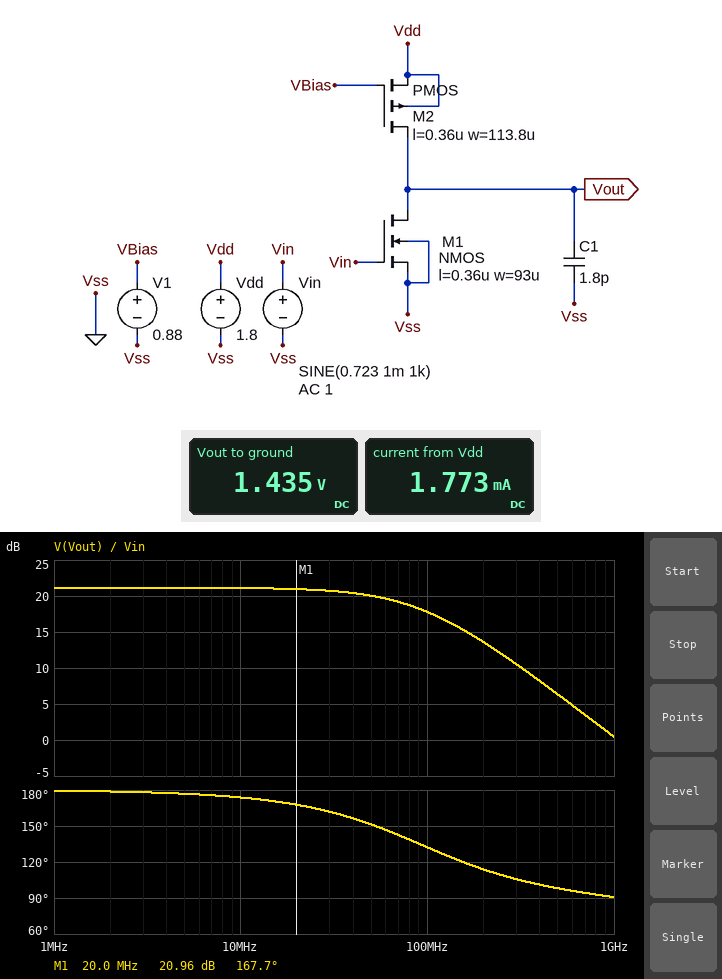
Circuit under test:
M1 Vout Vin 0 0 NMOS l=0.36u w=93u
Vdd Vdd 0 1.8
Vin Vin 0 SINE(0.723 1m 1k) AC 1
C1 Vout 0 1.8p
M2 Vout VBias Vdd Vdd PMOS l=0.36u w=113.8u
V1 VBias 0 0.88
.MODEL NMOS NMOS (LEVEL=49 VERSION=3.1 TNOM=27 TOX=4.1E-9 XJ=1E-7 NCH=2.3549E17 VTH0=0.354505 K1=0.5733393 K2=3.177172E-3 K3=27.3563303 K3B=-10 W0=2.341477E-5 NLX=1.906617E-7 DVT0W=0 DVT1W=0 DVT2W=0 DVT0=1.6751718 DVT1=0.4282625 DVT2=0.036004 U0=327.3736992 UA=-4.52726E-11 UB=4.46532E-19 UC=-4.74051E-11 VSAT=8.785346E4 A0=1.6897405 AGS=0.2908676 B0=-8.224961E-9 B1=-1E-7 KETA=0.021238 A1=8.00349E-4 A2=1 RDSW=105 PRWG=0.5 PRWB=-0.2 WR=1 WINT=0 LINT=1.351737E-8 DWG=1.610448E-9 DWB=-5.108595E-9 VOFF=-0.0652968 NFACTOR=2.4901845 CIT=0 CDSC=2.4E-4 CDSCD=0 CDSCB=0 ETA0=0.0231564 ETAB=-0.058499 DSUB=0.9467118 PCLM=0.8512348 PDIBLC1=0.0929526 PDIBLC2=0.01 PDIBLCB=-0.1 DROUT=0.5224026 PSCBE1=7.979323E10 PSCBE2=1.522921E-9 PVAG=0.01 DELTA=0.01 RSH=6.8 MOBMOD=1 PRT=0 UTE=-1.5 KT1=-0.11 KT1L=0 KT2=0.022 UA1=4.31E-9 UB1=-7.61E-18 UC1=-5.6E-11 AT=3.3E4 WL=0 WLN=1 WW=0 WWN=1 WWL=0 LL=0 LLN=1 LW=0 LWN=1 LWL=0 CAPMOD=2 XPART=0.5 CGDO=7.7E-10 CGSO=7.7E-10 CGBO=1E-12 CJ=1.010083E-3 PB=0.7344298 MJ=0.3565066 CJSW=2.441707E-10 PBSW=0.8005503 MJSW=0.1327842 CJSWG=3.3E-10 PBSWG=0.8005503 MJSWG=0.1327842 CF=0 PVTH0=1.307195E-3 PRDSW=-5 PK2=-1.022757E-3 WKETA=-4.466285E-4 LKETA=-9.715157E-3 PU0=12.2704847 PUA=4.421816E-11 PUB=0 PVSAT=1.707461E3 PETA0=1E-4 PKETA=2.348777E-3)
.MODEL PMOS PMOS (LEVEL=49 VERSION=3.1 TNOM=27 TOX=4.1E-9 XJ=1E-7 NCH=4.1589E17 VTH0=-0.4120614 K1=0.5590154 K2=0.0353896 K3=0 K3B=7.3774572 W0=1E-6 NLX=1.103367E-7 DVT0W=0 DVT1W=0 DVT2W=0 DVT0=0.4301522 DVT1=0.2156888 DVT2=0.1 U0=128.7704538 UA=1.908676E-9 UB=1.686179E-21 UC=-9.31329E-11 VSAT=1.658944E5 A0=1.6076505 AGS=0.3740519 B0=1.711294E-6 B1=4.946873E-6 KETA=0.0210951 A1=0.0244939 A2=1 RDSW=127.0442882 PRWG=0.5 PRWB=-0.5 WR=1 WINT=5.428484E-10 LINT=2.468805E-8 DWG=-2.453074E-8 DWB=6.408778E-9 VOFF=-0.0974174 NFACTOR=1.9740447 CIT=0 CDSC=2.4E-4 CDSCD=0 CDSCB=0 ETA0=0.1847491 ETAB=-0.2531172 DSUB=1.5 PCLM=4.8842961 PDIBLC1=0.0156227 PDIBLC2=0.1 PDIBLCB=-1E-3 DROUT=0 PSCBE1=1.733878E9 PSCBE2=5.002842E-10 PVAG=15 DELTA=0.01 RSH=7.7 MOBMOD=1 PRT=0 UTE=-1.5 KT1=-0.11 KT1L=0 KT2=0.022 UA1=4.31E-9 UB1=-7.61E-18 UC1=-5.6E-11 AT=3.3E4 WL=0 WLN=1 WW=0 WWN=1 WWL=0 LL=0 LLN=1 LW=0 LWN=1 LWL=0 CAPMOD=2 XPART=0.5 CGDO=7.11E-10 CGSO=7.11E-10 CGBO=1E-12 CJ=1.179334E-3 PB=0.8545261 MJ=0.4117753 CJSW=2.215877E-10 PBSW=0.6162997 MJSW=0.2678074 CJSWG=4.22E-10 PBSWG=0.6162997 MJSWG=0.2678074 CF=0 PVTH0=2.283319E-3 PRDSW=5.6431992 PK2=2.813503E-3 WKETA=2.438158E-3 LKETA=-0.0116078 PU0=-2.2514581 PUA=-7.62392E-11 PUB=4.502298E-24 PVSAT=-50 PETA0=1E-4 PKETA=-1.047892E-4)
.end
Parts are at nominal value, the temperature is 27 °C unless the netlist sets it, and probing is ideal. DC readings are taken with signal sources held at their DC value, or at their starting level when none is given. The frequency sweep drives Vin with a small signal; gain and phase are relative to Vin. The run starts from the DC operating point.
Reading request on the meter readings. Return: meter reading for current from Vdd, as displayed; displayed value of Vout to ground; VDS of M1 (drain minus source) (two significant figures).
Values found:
1.773 mA
1.435 V
1.4 V
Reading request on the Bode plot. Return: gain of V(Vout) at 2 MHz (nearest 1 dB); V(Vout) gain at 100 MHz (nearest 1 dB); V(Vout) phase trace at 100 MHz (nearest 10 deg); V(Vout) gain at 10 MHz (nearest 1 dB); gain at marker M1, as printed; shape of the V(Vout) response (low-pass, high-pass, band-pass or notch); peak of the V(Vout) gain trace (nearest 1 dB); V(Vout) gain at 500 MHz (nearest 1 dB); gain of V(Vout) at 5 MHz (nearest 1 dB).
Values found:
21 dB
18 dB
130 deg
21 dB
20.96 dB
low-pass
21 dB
6 dB
21 dB
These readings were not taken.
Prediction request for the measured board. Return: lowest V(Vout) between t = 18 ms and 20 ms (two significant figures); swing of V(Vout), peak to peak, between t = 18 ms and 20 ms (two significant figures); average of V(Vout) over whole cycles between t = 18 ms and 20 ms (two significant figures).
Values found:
1.4 V
23 mV
1.4 V
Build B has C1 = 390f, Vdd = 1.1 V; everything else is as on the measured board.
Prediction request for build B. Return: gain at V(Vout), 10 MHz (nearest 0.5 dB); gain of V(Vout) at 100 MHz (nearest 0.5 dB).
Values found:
-60.5 dB
-40.5 dB
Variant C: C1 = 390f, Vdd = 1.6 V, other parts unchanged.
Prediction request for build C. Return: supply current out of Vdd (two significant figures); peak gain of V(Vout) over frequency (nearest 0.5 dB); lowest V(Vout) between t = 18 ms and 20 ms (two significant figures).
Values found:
710 µA
-9.5 dB
60 mV
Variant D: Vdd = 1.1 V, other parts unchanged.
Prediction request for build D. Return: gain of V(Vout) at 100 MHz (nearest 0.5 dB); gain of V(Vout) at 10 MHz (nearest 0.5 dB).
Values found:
-40.5 dB
-60.5 dB
